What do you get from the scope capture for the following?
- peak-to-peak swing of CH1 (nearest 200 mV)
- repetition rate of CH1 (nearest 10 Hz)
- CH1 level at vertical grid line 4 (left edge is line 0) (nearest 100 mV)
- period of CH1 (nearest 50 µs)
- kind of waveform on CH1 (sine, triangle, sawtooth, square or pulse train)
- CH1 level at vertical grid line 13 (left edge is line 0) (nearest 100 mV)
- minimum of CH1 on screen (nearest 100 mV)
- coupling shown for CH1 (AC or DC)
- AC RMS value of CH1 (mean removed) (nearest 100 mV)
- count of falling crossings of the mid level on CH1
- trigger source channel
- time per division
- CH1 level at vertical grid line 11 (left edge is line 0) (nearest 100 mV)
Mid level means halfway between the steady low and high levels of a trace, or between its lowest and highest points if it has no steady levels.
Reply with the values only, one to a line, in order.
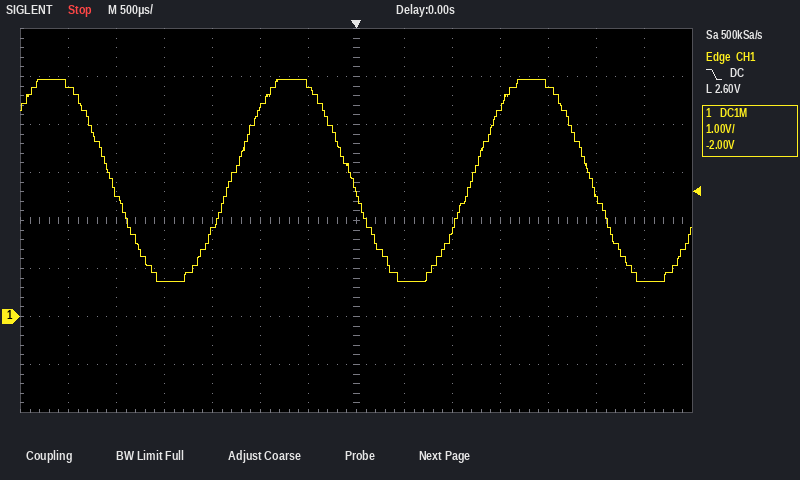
4.2 V
400 Hz
1.8 V
2.50 ms
sine
700 mV
700 mV
DC
1.5 V
3
CH1
500 µs
4.8 V
